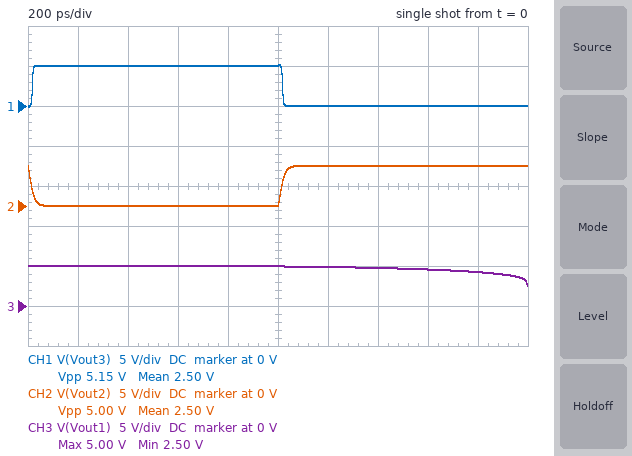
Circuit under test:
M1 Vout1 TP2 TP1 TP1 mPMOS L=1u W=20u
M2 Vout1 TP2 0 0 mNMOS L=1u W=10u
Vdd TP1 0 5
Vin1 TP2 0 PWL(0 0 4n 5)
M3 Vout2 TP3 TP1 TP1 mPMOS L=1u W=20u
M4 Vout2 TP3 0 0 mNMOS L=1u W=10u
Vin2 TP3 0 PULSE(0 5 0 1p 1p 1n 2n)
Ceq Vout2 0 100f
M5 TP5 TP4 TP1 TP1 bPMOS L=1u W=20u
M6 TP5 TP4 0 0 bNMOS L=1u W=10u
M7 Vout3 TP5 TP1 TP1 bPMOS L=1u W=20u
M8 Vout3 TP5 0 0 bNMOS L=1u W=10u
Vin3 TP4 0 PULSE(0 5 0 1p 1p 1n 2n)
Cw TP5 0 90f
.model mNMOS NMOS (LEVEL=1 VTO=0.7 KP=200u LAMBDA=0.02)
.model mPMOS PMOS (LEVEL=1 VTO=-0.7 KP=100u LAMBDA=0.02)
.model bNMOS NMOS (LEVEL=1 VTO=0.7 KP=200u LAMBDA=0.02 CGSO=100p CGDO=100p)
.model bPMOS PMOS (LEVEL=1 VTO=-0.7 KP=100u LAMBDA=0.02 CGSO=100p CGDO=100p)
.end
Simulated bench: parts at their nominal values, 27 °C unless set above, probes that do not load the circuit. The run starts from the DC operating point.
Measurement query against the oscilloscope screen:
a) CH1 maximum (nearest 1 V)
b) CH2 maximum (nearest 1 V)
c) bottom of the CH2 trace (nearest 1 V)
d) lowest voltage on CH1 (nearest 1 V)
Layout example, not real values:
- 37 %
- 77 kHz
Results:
- 5 V
- 5 V
- 0 V
- 0 V
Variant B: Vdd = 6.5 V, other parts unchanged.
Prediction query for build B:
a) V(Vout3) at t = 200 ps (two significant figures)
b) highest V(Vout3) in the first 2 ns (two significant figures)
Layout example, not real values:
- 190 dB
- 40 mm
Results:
- 6.5 V
- 6.6 V
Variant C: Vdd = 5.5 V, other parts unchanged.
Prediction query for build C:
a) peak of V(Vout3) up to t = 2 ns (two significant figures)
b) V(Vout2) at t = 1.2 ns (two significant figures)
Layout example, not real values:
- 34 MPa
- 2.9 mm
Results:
- 5.6 V
- 5.5 V
